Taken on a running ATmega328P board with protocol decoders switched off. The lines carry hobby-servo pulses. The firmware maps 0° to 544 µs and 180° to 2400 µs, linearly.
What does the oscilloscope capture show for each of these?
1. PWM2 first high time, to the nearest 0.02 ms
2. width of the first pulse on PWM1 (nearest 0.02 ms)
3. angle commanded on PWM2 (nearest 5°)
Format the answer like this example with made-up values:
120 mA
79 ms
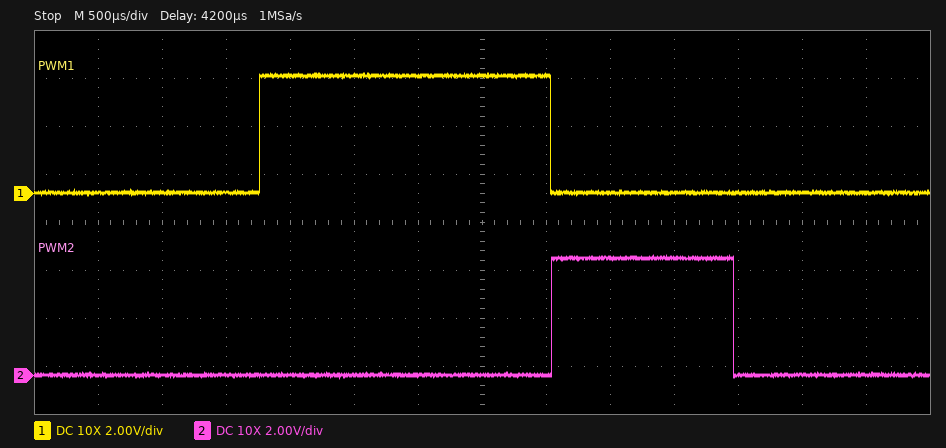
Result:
1.42 ms
2.28 ms
85°
